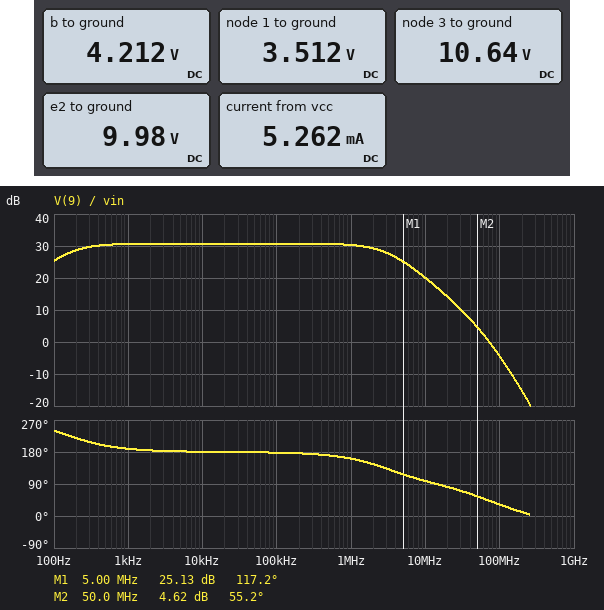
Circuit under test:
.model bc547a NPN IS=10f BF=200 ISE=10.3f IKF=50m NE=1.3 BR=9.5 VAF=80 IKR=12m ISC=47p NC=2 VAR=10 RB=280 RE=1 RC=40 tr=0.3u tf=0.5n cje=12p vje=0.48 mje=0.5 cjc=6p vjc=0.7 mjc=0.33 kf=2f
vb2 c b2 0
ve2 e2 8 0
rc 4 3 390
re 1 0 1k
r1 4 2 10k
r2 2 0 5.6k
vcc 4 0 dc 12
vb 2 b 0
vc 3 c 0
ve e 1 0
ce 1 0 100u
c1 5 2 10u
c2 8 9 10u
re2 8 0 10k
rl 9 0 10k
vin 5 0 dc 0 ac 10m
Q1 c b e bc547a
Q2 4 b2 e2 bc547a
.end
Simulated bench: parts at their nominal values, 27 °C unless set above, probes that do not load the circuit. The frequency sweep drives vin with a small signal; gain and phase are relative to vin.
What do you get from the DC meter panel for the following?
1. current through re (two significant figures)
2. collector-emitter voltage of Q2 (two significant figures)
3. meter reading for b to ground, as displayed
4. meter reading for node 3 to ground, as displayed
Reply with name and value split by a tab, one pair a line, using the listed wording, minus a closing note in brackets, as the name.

current through re	3.5 mA
collector-emitter voltage of Q2	2.0 V
meter reading for b to ground, as displayed	4.212 V
meter reading for node 3 to ground, as displayed	10.64 V
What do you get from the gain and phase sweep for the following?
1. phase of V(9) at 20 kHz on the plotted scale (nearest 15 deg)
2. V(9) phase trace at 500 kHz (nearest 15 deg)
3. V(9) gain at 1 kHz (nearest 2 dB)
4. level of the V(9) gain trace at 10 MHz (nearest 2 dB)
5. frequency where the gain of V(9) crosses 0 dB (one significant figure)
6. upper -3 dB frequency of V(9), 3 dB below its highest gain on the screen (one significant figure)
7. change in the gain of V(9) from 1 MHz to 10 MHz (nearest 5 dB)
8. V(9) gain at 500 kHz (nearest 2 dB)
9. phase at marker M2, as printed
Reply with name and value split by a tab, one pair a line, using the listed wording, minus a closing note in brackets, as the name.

phase of V(9) at 20 kHz on the plotted scale	180 deg
V(9) phase trace at 500 kHz	165 deg
V(9) gain at 1 kHz	30 dB
level of the V(9) gain trace at 10 MHz	20 dB
frequency where the gain of V(9) crosses 0 dB	70 MHz
upper -3 dB frequency of V(9), 3 dB below its highest gain on the screen	3 MHz
change in the gain of V(9) from 1 MHz to 10 MHz	-10 dB
V(9) gain at 500 kHz	30 dB
phase at marker M2, as printed	55.2 deg
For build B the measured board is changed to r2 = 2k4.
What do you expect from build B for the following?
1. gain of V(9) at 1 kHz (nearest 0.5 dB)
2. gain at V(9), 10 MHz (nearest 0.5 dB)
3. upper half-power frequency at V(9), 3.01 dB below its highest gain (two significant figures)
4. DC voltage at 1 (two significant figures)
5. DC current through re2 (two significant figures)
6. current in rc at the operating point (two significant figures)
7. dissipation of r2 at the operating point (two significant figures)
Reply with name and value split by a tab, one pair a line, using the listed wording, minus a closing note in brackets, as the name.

gain of V(9) at 1 kHz	26.0 dB
gain at V(9), 10 MHz	18.5 dB
upper half-power frequency at V(9), 3.01 dB below its highest gain	4.9 MHz
DC voltage at 1	1.6 V
DC current through re2	1.1 mA
current in rc at the operating point	1.6 mA
dissipation of r2 at the operating point	2.2 mW
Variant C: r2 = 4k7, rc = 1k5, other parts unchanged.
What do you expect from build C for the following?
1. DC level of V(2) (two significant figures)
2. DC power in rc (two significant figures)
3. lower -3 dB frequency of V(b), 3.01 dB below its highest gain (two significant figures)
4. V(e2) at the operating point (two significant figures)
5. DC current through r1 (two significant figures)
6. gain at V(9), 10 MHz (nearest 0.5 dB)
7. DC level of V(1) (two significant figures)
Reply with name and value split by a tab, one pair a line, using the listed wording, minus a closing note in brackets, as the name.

DC level of V(2)	3.8 V
DC power in rc	14 mW
lower -3 dB frequency of V(b), 3.01 dB below its highest gain	5.6 Hz
V(e2) at the operating point	6.8 V
DC current through r1	820 µA
gain at V(9), 10 MHz	22.5 dB
DC level of V(1)	3.1 V
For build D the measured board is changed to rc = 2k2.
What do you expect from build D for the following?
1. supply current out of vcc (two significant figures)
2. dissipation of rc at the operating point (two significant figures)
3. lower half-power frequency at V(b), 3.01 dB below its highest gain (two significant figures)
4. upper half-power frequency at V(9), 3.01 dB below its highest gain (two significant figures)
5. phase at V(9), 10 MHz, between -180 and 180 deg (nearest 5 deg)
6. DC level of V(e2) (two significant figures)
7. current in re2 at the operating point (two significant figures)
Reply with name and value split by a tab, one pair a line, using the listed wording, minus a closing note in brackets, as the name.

supply current out of vcc	4.6 mA
dissipation of rc at the operating point	27 mW
lower half-power frequency at V(b), 3.01 dB below its highest gain	5.1 Hz
upper half-power frequency at V(9), 3.01 dB below its highest gain	470 kHz
phase at V(9), 10 MHz, between -180 and 180 deg	85 deg
DC level of V(e2)	3.7 V
current in re2 at the operating point	370 µA
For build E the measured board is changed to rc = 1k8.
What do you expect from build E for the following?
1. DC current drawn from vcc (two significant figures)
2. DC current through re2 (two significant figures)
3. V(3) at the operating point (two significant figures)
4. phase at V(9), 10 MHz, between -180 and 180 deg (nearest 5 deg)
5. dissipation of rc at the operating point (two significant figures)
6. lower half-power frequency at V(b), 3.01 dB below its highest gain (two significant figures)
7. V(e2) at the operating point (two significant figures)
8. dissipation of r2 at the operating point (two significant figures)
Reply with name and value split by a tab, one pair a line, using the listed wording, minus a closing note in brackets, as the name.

DC current drawn from vcc	4.8 mA
DC current through re2	510 µA
V(3) at the operating point	5.7 V
phase at V(9), 10 MHz, between -180 and 180 deg	85 deg
dissipation of rc at the operating point	22 mW
lower half-power frequency at V(b), 3.01 dB below its highest gain	5.1 Hz
V(e2) at the operating point	5.1 V
dissipation of r2 at the operating point	3.2 mW
